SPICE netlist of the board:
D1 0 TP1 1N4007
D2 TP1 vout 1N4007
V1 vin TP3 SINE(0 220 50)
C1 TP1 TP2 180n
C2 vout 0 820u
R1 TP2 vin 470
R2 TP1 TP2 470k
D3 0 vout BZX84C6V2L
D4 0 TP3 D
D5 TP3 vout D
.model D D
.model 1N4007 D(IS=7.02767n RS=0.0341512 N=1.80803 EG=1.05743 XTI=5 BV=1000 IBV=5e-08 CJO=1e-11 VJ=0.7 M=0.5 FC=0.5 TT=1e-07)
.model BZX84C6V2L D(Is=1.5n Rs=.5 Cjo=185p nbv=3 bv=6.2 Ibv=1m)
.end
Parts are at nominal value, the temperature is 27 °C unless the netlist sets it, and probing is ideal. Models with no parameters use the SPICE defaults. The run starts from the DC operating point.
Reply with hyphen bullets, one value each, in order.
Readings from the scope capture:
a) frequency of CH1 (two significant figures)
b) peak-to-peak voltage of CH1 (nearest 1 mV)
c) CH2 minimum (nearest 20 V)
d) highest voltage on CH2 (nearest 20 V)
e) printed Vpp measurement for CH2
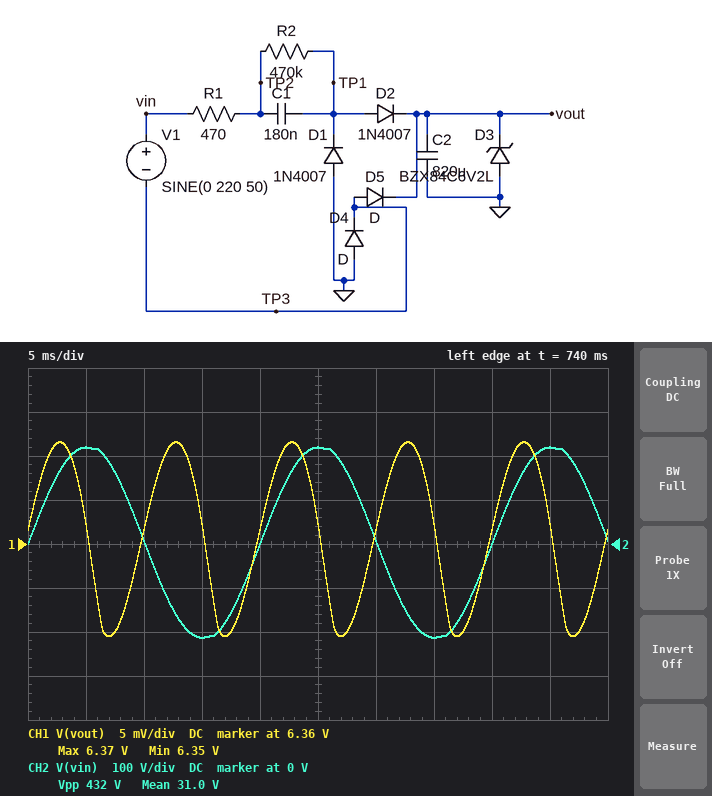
- 100 Hz
- 22 mV
- -220 V
- 220 V
- 432 V
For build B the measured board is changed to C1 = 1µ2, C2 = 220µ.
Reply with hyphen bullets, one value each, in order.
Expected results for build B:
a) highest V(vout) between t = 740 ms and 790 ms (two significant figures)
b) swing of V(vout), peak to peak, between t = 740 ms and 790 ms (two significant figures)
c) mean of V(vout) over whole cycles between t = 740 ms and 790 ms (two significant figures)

- 6.6 V
- 200 mV
- 6.5 V
